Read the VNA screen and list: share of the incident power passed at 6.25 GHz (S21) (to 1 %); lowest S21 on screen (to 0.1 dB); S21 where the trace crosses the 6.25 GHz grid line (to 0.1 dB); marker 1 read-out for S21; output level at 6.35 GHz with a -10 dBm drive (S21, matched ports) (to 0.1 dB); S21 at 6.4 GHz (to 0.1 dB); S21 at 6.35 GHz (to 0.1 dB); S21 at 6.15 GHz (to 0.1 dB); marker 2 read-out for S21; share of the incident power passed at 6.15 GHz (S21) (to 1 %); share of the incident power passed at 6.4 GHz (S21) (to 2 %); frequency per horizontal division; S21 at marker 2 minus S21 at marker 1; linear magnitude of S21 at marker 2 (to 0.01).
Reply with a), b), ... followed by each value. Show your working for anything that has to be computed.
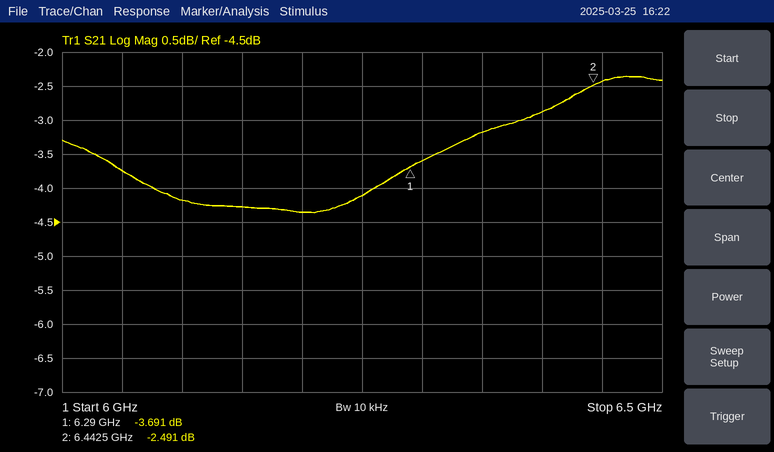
a) 10^(-4.1/10) ≈ 39 %
b) -4.4 dB
c) -4.1 dB
d) -3.691 dB
e) -10 dBm + (-3.2 dB) = -13.2 dBm
f) -2.9 dB
g) -3.2 dB
h) -4.3 dB
i) -2.491 dB
j) 10^(-4.3/10) ≈ 37 %
k) 10^(-2.9/10) ≈ 51.3 %, so 52 % to the nearest 2 %
l) 50 MHz
m) -2.491 − (-3.691) = 1.200 dB
n) 10^(-2.491/20) ≈ 0.75
